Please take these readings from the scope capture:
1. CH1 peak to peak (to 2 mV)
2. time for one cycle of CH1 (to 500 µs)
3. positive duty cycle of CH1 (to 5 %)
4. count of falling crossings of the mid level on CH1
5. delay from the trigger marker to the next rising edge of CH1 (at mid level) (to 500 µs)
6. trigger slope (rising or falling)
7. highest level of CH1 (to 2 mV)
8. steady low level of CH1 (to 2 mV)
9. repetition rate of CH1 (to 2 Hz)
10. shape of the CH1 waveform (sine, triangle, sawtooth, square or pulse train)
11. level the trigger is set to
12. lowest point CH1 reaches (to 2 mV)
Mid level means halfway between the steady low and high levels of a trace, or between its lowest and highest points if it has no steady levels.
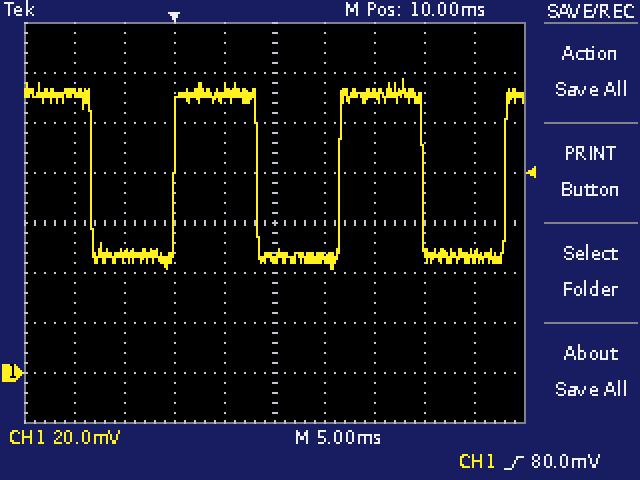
76 mV
16.5 ms
50 %
3
16.5 ms
rising
118 mV
46 mV
60 Hz
square
80.0 mV
42 mV
